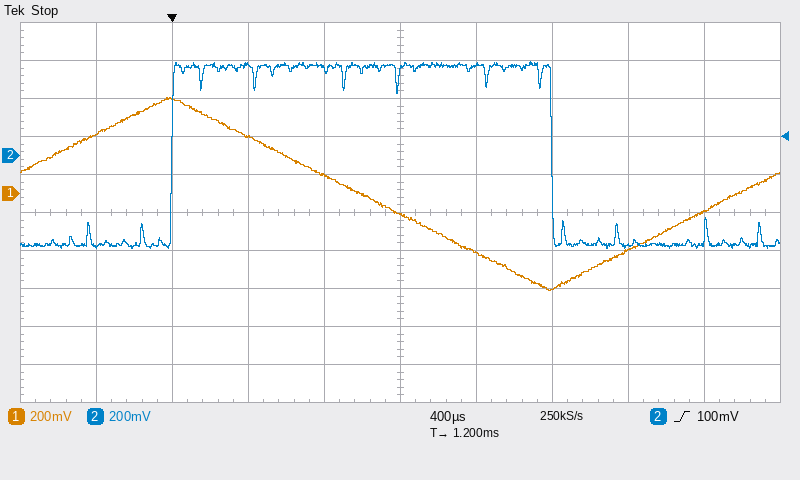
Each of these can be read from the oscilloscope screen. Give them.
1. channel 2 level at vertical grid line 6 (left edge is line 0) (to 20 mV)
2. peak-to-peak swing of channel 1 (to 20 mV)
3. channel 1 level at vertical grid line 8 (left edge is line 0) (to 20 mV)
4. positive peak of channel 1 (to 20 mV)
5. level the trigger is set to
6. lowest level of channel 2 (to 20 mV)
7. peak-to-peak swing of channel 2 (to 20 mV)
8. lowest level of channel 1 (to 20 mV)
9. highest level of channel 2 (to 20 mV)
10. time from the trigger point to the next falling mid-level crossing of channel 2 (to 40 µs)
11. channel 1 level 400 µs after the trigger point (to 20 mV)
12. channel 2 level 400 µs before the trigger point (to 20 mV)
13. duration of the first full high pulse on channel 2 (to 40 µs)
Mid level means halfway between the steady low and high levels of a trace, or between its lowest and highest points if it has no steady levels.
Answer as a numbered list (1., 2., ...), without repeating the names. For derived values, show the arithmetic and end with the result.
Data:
1. 480 mV
2. 500 mV − (-520 mV) = 1.02 V
3. -300 mV
4. 500 mV
5. 100 mV
6. -480 mV
7. 500 mV − (-480 mV) = 980 mV
8. -520 mV
9. 500 mV
10. 2.00 ms
11. 300 mV
12. -480 mV
13. 2.00 ms
